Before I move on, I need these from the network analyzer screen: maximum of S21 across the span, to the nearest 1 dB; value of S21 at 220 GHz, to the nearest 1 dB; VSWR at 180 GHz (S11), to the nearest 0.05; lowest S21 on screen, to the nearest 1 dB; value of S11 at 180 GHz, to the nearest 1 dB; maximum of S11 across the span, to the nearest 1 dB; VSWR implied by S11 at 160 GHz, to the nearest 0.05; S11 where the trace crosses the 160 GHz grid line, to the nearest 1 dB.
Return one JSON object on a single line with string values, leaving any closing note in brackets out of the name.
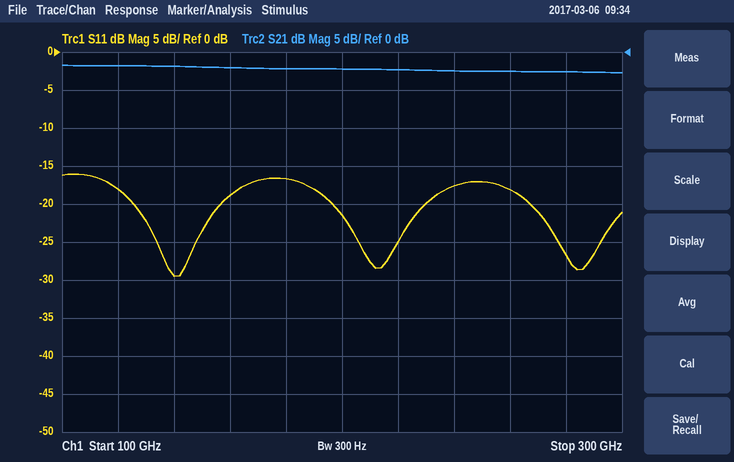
{"maximum of S21 across the span, to the nearest 1 dB": "-2 dB", "value of S21 at 220 GHz, to the nearest 1 dB": "-2 dB", "VSWR at 180 GHz (S11), to the nearest 0.05": "1.35", "lowest S21 on screen, to the nearest 1 dB": "-3 dB", "value of S11 at 180 GHz, to the nearest 1 dB": "-17 dB", "maximum of S11 across the span, to the nearest 1 dB": "-16 dB", "VSWR implied by S11 at 160 GHz, to the nearest 0.05": "1.25", "S11 where the trace crosses the 160 GHz grid line, to the nearest 1 dB": "-19 dB"}
